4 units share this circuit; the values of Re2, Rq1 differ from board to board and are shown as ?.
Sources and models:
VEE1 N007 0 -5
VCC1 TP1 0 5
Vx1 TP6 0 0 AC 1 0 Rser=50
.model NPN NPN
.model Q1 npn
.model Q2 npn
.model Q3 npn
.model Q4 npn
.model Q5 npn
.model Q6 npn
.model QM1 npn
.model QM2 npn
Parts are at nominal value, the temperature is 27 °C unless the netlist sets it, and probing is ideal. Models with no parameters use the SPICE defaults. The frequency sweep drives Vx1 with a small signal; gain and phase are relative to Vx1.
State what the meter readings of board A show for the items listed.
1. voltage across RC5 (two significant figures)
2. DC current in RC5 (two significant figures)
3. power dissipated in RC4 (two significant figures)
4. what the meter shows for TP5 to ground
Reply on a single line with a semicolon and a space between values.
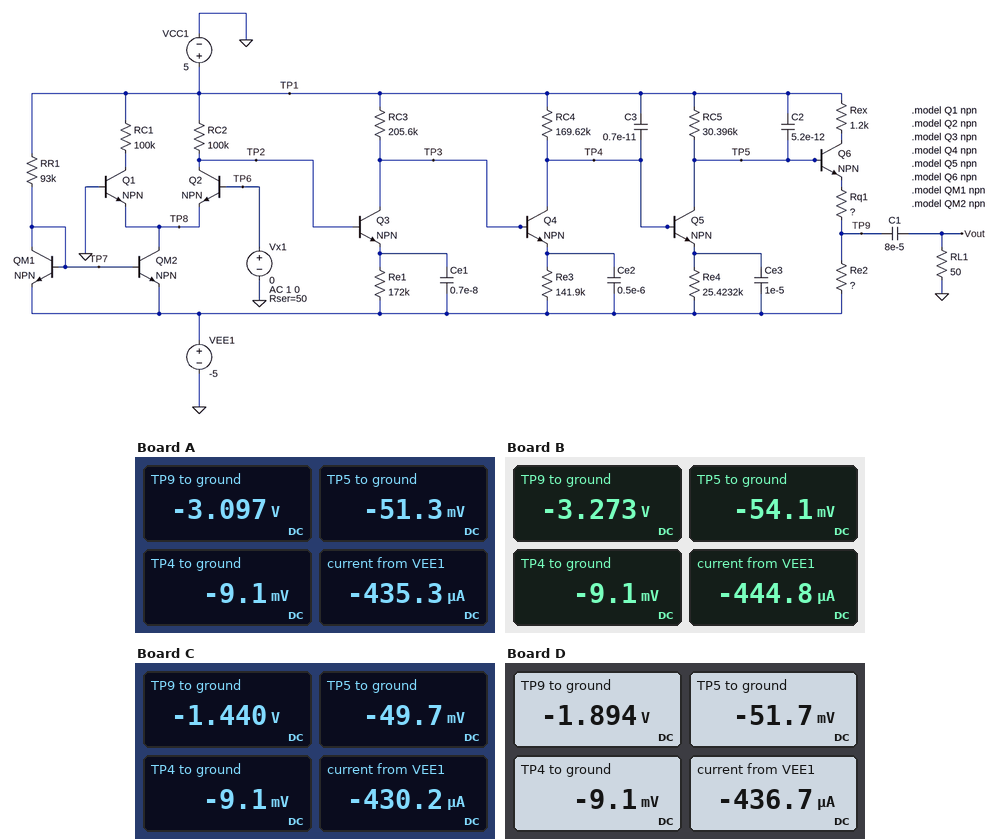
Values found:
5.1 V; 170 µA; 150 µW; -51.3 mV
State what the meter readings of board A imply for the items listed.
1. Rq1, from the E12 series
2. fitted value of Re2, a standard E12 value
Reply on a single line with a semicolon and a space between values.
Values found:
150 kΩ; 120 kΩ
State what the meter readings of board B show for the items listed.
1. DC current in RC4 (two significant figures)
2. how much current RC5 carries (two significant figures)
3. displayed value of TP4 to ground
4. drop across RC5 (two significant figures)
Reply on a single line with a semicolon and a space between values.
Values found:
30 µA; 170 µA; -9.1 mV; 5.1 V
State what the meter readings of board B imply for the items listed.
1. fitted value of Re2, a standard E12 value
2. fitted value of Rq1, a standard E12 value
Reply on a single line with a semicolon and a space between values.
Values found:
68 kΩ; 100 kΩ
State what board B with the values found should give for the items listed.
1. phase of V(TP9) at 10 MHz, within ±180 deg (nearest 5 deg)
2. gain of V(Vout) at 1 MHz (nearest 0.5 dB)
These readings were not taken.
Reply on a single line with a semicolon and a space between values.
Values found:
-165 deg; 64.5 dB
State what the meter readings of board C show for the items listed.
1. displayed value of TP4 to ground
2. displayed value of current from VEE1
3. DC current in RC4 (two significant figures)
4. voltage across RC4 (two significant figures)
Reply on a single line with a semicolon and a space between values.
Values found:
-9.1 mV; -430.2 µA; 30 µA; 5.0 V
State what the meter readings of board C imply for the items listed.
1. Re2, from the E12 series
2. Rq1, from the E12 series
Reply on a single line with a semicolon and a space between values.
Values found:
330 kΩ; 68 kΩ
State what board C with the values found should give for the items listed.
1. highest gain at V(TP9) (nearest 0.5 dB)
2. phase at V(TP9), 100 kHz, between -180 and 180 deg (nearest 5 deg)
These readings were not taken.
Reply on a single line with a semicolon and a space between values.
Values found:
72.0 dB; -5 deg
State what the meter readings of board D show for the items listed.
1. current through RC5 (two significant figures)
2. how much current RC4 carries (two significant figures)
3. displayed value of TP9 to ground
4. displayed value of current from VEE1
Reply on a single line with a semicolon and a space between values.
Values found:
170 µA; 30 µA; -1.894 V; -436.7 µA
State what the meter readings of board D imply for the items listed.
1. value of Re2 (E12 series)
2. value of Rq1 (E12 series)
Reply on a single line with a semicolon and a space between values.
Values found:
180 kΩ; 68 kΩ
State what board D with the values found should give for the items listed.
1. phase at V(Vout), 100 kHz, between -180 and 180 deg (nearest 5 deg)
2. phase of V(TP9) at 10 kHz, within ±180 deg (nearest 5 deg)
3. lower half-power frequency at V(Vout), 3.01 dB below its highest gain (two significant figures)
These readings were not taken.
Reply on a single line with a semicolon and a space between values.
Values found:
-5 deg; 35 deg; 7.7 kHz
